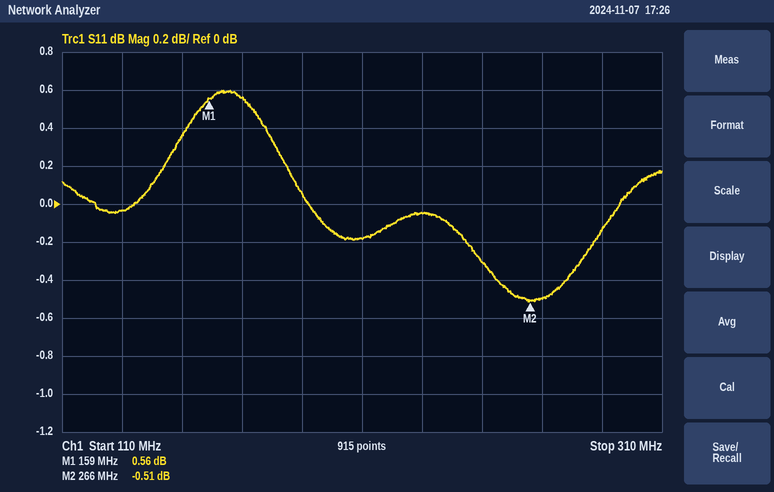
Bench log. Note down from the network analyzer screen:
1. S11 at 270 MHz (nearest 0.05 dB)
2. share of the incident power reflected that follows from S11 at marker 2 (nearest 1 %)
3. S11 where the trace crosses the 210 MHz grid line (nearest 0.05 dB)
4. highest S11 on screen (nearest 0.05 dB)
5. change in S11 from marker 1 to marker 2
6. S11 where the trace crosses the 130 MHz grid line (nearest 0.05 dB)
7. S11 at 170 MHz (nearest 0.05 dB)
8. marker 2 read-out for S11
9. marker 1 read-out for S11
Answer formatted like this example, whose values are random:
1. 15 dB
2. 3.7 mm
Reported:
1. -0.50 dB
2. 89 %
3. -0.20 dB
4. 0.60 dB
5. -1.07 dB
6. -0.05 dB
7. 0.55 dB
8. -0.51 dB
9. 0.56 dB
